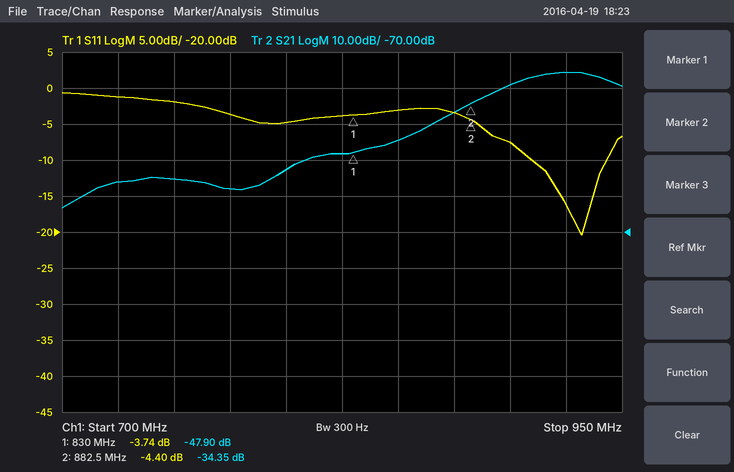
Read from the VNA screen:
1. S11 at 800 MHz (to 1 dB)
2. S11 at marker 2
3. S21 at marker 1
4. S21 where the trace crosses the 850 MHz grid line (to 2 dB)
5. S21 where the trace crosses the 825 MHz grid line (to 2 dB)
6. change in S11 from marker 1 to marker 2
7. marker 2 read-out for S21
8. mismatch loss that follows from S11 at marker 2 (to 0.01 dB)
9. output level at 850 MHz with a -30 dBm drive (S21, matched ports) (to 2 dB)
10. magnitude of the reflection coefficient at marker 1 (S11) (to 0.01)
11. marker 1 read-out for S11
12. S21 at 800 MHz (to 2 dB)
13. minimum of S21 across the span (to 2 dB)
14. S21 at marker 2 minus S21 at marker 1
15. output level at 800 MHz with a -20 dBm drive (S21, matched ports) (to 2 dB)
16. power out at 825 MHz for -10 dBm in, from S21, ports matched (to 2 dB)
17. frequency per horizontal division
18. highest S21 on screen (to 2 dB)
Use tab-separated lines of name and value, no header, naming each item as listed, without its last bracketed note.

S11 at 800 MHz	-5 dB
S11 at marker 2	-4.40 dB
S21 at marker 1	-47.90 dB
S21 where the trace crosses the 850 MHz grid line	-44 dB
S21 where the trace crosses the 825 MHz grid line	-48 dB
change in S11 from marker 1 to marker 2	-0.66 dB
marker 2 read-out for S21	-34.35 dB
mismatch loss that follows from S11 at marker 2	1.96 dB
output level at 850 MHz with a -30 dBm drive (S21, matched ports)	-74 dBm
magnitude of the reflection coefficient at marker 1 (S11)	0.65
marker 1 read-out for S11	-3.74 dB
S21 at 800 MHz	-52 dB
minimum of S21 across the span	-64 dB
S21 at marker 2 minus S21 at marker 1	13.55 dB
output level at 800 MHz with a -20 dBm drive (S21, matched ports)	-72 dBm
power out at 825 MHz for -10 dBm in, from S21, ports matched	-58 dBm
frequency per horizontal division	25 MHz
highest S21 on screen	-26 dB
